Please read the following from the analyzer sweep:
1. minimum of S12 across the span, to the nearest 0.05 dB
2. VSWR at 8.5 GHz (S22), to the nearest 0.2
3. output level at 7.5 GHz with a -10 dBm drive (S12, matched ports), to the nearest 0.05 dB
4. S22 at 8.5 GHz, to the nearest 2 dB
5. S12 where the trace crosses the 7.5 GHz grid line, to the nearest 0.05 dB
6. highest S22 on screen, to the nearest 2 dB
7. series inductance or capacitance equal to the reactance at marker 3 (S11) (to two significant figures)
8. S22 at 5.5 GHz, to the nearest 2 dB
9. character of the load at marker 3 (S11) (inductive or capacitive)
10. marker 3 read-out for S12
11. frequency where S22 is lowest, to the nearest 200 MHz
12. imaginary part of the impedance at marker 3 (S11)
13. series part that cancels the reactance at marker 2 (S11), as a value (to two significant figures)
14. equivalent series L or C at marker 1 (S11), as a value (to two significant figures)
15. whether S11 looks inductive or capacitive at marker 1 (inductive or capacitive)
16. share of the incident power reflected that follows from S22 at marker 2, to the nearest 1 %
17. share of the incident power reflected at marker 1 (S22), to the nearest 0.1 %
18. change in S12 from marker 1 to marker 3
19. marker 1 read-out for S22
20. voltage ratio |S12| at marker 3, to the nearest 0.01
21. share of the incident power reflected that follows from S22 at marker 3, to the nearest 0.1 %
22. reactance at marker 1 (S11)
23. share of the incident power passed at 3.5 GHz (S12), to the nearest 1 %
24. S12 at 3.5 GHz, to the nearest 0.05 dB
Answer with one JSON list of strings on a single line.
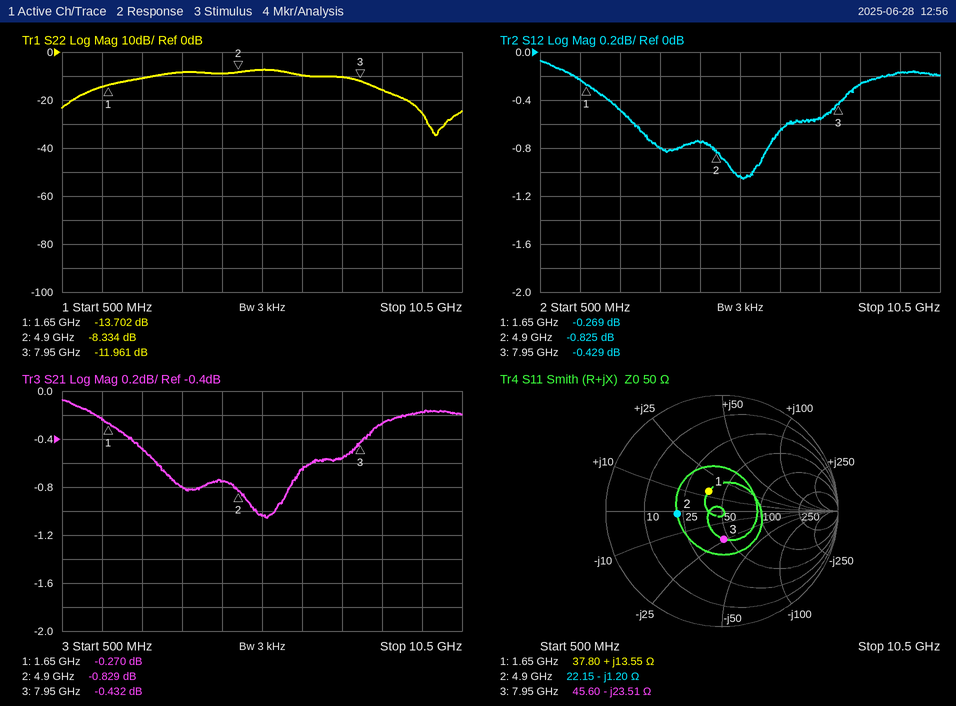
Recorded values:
["-1.05 dB", "1.4", "-10.55 dBm", "-16 dB", "-0.55 dB", "-8 dB", "850 fF", "-8 dB", "capacitive", "-0.429 dB", "9.8 GHz", "-23.51 Ω", "39 pH", "1.3 nH", "inductive", "15 %", "4.3 %", "-0.160 dB", "-13.702 dB", "0.95", "6.4 %", "+13.55 Ω", "83 %", "-0.80 dB"]
